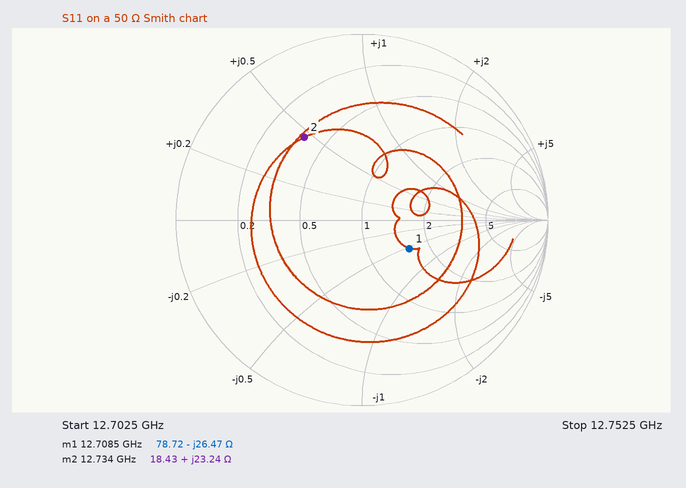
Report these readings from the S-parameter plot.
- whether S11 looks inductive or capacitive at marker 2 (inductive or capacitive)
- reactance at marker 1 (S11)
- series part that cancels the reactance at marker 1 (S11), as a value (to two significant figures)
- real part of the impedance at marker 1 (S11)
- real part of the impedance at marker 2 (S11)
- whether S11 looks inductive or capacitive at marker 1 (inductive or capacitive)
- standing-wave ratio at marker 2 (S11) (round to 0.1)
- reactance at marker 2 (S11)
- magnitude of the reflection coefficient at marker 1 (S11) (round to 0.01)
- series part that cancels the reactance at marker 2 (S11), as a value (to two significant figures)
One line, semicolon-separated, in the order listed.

inductive; -26.47 Ω; 330 pH; 78.72 Ω; 18.43 Ω; capacitive; 3.4; +23.24 Ω; 0.30; 540 fF
